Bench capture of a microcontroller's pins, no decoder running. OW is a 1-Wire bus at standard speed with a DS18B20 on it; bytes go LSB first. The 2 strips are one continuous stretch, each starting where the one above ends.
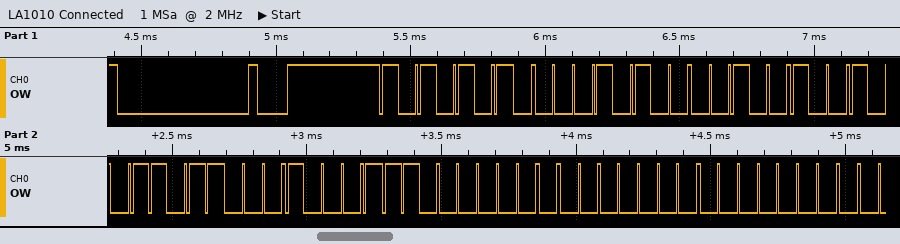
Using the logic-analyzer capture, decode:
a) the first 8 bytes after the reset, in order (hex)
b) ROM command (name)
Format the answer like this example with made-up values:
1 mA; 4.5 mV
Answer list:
55 28 24 D9 88 03 00 00; Match ROM
